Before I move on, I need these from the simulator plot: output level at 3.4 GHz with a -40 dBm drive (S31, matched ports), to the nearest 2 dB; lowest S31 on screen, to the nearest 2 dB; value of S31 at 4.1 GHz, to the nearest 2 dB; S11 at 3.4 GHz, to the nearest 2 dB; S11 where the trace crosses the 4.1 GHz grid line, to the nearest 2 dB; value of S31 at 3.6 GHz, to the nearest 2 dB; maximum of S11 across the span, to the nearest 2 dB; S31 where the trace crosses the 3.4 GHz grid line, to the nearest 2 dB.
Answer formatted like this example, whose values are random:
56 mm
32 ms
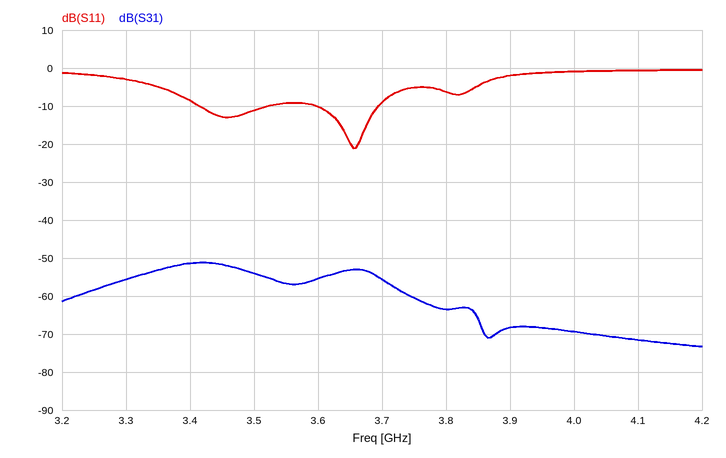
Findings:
-92 dBm
-74 dB
-72 dB
-8 dB
0 dB
-56 dB
0 dB
-52 dB
